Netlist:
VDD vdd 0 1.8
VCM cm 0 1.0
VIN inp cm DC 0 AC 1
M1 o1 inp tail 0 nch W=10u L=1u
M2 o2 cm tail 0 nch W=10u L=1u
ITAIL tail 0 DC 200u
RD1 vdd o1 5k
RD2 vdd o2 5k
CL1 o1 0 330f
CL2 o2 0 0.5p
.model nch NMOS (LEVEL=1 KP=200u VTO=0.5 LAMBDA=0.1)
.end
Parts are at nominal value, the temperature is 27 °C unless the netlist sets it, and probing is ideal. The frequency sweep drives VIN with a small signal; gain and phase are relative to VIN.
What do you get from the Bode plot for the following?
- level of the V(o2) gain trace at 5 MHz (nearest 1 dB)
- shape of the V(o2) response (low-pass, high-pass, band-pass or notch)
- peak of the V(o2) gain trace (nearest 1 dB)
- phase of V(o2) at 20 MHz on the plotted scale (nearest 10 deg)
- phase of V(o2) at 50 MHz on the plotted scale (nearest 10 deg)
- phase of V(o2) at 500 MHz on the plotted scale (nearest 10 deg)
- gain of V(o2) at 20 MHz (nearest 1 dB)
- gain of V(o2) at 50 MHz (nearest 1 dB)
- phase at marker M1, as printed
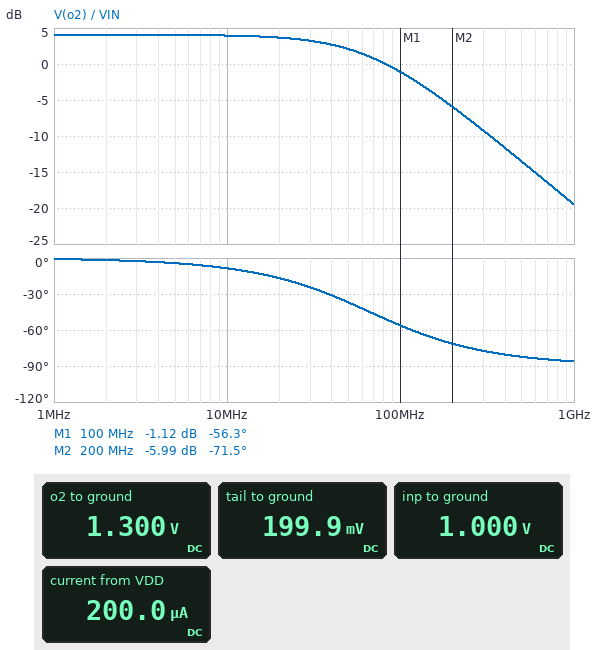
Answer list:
4 dB
low-pass
4 dB
-20 deg
-40 deg
-80 deg
4 dB
2 dB
-56.3 deg
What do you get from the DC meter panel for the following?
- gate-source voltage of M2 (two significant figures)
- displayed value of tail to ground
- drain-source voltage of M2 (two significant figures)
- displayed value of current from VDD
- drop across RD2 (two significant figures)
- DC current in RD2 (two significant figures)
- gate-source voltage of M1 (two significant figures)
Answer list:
800 mV
199.9 mV
1.1 V
200.0 µA
500 mV
100 µA
800 mV
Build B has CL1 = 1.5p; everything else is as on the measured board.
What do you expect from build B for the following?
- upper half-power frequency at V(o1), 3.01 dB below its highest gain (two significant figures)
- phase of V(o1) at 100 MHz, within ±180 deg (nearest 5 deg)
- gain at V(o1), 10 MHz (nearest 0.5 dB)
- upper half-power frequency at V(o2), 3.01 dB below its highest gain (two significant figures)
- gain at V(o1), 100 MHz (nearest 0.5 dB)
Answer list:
22 MHz
105 deg
3.0 dB
68 MHz
-9.5 dB
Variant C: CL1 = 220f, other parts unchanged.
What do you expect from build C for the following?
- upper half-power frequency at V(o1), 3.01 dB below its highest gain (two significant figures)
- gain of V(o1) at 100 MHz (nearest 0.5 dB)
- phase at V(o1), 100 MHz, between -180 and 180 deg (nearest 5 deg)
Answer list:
150 MHz
2.5 dB
145 deg
